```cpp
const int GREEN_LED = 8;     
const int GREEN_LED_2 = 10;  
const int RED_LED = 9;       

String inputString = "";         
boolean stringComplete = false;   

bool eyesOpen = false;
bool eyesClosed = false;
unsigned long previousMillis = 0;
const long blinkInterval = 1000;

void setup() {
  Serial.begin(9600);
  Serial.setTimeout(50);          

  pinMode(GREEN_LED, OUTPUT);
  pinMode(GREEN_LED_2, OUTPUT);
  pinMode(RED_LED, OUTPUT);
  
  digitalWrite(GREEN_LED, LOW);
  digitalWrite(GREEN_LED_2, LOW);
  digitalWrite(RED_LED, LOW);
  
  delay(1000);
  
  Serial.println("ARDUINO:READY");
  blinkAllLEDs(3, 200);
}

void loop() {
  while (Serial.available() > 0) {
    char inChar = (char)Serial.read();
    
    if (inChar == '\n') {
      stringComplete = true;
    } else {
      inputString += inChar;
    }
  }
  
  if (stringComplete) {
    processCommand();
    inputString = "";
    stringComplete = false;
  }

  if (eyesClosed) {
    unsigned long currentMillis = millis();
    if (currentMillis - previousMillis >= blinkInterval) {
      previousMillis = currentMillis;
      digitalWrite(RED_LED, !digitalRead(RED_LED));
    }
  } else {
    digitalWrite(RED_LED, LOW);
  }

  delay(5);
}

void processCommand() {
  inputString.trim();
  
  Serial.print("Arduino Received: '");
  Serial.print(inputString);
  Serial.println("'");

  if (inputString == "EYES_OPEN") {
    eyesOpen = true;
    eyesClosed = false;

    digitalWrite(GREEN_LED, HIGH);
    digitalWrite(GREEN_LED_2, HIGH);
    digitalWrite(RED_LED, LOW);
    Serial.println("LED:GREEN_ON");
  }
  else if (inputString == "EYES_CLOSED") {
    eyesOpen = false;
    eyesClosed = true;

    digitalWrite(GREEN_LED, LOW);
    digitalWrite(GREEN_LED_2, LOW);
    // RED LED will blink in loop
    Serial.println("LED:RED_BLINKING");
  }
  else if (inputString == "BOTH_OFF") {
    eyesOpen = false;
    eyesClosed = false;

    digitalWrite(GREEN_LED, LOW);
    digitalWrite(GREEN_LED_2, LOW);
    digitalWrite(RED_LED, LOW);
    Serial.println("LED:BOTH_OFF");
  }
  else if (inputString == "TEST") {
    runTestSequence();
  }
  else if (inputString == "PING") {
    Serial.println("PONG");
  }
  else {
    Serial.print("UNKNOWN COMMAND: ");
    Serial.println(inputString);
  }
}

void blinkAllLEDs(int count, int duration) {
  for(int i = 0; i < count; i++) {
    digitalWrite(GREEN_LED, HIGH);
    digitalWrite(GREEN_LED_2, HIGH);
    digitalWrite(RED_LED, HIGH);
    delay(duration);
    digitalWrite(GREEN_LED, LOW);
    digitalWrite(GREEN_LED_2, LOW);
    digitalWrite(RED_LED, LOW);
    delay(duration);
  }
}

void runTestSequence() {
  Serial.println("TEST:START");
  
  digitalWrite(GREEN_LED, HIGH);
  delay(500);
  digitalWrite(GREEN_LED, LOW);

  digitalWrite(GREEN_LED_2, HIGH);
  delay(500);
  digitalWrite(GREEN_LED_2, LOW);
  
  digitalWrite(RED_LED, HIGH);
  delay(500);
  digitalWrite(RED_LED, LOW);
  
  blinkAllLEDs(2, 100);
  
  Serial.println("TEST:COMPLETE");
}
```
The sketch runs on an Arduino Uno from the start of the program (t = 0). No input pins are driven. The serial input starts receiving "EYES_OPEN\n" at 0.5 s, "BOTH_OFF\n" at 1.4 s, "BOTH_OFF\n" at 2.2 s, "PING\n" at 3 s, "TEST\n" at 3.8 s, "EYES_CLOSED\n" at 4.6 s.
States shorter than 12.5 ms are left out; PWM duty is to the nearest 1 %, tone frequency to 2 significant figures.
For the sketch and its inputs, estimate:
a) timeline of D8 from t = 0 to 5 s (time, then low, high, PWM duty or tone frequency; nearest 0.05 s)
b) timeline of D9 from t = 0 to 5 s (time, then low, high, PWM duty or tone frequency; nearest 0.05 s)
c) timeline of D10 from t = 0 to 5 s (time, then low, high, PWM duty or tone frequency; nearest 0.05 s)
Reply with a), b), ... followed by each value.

a) 0 s low; 1 s high; 1.2 s low; 1.4 s high; 1.6 s low; 1.8 s high; 2 s low; 3.8 s high; 4.3 s low
b) 0 s low; 1 s high; 1.2 s low; 1.4 s high; 1.6 s low; 1.8 s high; 2 s low; 4.8 s high
c) 0 s low; 1 s high; 1.2 s low; 1.4 s high; 1.6 s low; 1.8 s high; 2 s low; 4.3 s high; 4.8 s low
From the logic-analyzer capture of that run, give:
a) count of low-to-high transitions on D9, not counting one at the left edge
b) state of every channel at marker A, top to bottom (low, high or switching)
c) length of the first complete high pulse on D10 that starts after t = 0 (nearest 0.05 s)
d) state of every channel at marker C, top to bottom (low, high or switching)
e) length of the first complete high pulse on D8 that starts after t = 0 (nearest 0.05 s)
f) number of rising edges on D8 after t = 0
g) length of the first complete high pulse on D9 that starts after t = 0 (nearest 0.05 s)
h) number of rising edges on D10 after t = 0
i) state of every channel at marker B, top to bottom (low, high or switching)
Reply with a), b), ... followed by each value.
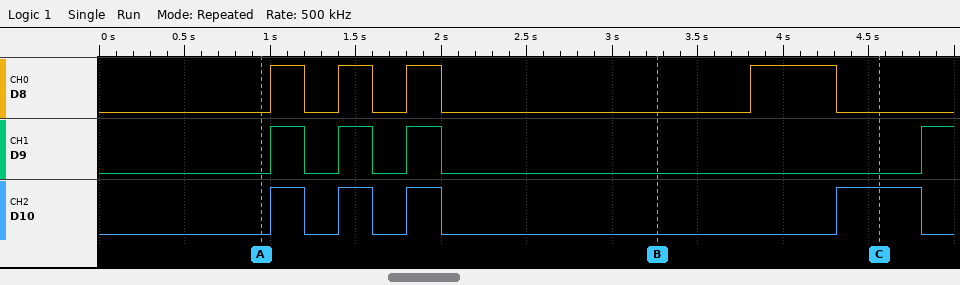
a) 4
b) D8 low, D9 low, D10 low
c) 0.20 s
d) D8 low, D9 low, D10 high
e) 0.20 s
f) 4
g) 0.20 s
h) 4
i) D8 low, D9 low, D10 low
